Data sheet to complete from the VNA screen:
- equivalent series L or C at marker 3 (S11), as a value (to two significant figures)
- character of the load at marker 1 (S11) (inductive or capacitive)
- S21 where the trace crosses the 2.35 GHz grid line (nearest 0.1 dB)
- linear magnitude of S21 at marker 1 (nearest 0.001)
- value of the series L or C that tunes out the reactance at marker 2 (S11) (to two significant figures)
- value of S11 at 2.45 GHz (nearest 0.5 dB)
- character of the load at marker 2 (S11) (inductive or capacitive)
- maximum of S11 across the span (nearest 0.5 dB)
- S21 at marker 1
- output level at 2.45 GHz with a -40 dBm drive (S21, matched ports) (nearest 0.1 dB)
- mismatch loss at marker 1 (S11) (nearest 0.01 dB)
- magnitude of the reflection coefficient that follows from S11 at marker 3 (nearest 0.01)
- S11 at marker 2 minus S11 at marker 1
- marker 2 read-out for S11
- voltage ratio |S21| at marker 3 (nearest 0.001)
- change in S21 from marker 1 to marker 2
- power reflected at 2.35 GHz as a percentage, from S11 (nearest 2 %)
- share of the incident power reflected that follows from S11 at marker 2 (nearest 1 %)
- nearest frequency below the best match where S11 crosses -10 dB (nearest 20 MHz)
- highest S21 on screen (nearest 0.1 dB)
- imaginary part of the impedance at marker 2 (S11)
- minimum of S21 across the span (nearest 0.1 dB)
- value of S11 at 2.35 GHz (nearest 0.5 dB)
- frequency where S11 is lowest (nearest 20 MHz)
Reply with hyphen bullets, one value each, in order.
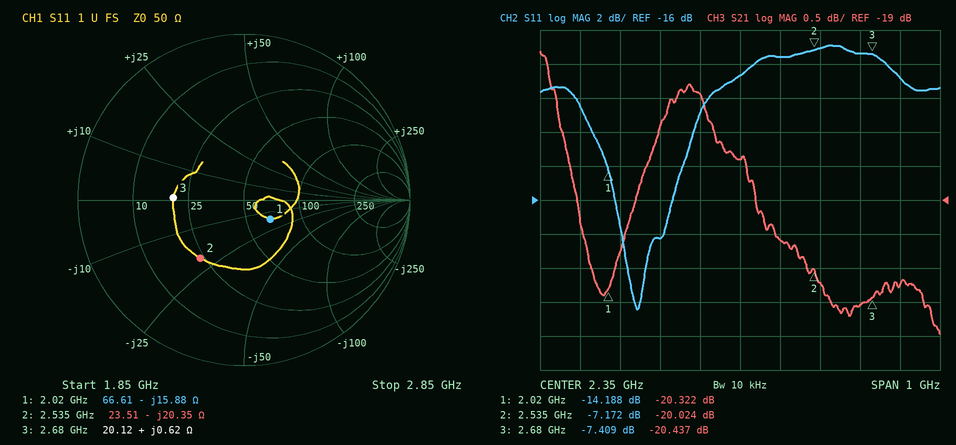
- 37 pH
- capacitive
- -18.4 dB
- 0.096
- 1.3 nH
- -7.5 dB
- capacitive
- -7.0 dB
- -20.322 dB
- -59.6 dBm
- 0.17 dB
- 0.43
- 7.016 dB
- -7.172 dB
- 0.095
- 0.298 dB
- 14 %
- 19 %
- 1.94 GHz
- -16.8 dB
- -20.35 Ω
- -21.0 dB
- -8.5 dB
- 2.10 GHz
